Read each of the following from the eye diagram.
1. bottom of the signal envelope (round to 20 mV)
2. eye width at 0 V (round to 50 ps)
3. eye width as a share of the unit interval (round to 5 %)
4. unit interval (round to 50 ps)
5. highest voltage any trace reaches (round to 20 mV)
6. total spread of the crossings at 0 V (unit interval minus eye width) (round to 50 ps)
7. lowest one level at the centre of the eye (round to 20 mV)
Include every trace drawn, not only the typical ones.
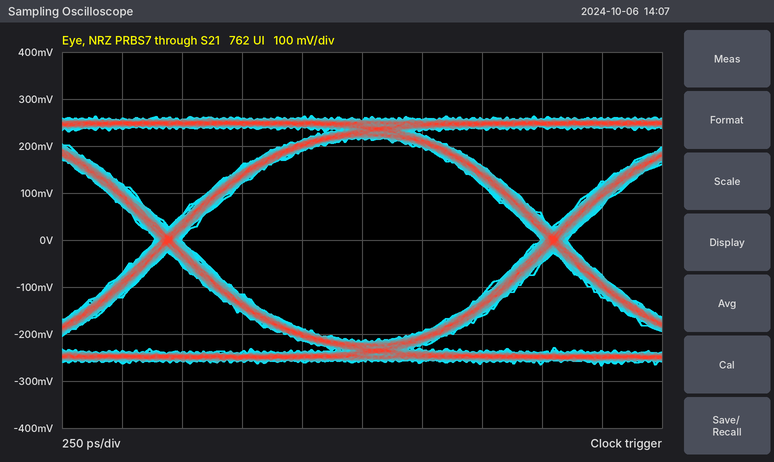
-260 mV
1.50 ns
95 %
1.60 ns
260 mV
100 ps
220 mV
